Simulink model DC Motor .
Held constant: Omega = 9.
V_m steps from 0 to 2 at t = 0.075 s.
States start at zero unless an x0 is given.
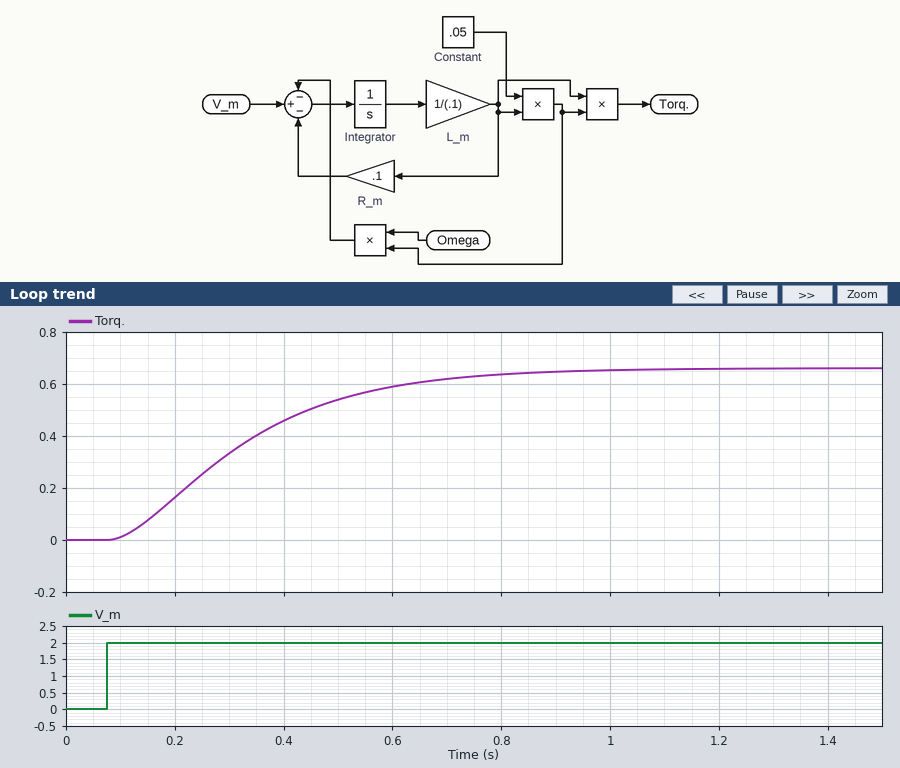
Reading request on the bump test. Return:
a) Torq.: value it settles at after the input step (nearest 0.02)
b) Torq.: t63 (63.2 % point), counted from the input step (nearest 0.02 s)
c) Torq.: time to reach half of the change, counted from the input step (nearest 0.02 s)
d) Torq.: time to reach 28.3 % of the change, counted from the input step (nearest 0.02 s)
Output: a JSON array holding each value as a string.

["0.66", "0.28 s", "0.22 s", "0.14 s"]
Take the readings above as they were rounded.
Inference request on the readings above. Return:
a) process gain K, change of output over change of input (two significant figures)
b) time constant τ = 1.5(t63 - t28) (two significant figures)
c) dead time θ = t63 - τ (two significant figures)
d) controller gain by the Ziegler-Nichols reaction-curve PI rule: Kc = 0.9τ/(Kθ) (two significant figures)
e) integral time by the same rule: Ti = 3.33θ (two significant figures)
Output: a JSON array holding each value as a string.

["0.33", "0.21 s", "0.070 s", "8.2", "0.23 s"]
